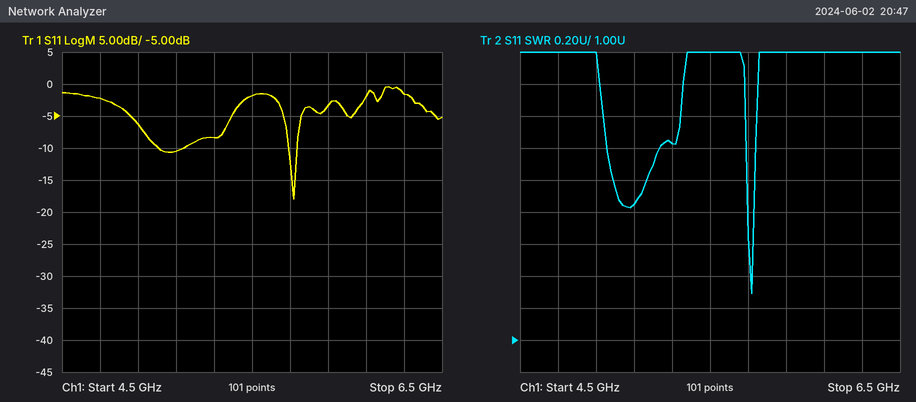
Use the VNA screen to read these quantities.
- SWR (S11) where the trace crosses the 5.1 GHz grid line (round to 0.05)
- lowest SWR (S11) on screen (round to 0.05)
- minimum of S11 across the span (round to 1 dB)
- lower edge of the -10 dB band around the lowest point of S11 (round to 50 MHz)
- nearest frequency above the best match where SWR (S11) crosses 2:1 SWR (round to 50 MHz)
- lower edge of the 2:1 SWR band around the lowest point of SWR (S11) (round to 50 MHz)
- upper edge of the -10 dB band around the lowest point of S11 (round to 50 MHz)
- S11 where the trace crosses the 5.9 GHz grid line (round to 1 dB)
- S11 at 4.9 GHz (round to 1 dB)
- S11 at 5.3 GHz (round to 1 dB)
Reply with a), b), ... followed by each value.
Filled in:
a) 1.85
b) 1.30
c) -18 dB
d) 5.70 GHz
e) 5.75 GHz
f) 5.70 GHz
g) 5.75 GHz
h) -3 dB
i) -6 dB
j) -8 dB
